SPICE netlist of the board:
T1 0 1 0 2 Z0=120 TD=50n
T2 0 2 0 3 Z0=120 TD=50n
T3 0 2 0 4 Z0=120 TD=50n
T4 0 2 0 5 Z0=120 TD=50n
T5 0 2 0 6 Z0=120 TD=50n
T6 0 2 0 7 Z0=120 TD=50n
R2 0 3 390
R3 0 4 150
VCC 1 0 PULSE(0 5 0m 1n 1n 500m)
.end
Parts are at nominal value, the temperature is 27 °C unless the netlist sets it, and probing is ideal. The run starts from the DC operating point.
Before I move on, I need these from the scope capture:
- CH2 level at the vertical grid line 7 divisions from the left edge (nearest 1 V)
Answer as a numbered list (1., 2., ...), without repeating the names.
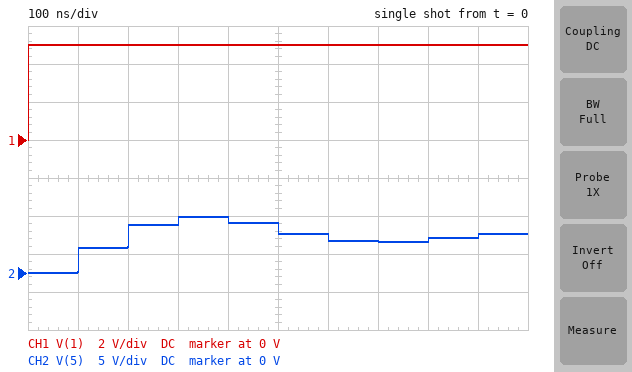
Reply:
1. 4 V
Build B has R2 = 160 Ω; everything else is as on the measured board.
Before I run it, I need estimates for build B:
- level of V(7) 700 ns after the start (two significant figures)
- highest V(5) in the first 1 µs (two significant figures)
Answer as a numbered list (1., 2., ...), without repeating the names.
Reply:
1. 4.6 V
2. 6.6 V
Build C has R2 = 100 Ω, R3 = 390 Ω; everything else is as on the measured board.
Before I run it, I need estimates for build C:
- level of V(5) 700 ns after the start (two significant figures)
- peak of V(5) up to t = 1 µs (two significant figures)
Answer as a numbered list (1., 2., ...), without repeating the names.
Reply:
1. 4.4 V
2. 6.8 V
